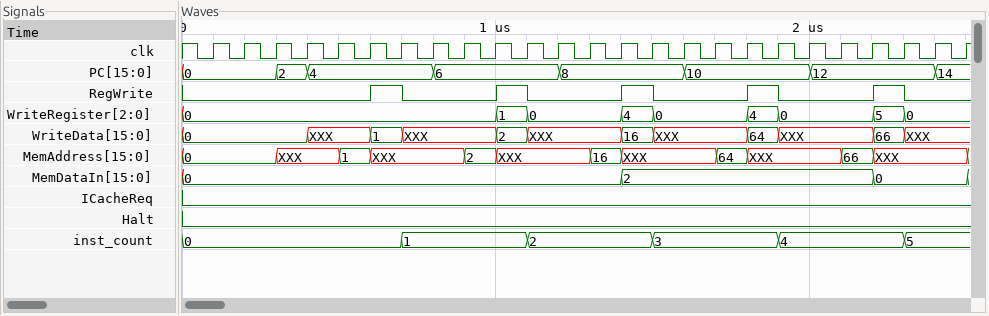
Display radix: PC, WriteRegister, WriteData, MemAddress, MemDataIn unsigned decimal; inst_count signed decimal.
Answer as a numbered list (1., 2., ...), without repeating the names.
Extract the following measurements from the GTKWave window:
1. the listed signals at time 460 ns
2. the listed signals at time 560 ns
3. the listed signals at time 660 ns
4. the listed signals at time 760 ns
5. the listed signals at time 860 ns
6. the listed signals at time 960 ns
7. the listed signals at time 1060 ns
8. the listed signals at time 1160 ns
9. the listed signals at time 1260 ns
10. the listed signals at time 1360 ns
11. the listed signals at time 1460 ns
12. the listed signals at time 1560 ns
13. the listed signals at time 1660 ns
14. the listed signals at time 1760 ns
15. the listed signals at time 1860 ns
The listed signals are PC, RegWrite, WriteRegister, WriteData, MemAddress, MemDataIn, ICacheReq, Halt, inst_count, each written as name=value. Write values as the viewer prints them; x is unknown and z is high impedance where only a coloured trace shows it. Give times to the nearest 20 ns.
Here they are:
1. PC=4, RegWrite=0, WriteRegister=0, WriteData=XXX, MemAddress=XXX, MemDataIn=0, ICacheReq=0, Halt=0, inst_count=0
2. PC=4, RegWrite=0, WriteRegister=0, WriteData=XXX, MemAddress=1, MemDataIn=0, ICacheReq=0, Halt=0, inst_count=0
3. PC=4, RegWrite=1, WriteRegister=0, WriteData=1, MemAddress=XXX, MemDataIn=0, ICacheReq=0, Halt=0, inst_count=0
4. PC=4, RegWrite=0, WriteRegister=0, WriteData=XXX, MemAddress=XXX, MemDataIn=0, ICacheReq=0, Halt=0, inst_count=1
5. PC=6, RegWrite=0, WriteRegister=0, WriteData=XXX, MemAddress=XXX, MemDataIn=0, ICacheReq=0, Halt=0, inst_count=1
6. PC=6, RegWrite=0, WriteRegister=0, WriteData=XXX, MemAddress=2, MemDataIn=0, ICacheReq=0, Halt=0, inst_count=1
7. PC=6, RegWrite=1, WriteRegister=1, WriteData=2, MemAddress=XXX, MemDataIn=0, ICacheReq=0, Halt=0, inst_count=1
8. PC=6, RegWrite=0, WriteRegister=0, WriteData=XXX, MemAddress=XXX, MemDataIn=0, ICacheReq=0, Halt=0, inst_count=2
9. PC=8, RegWrite=0, WriteRegister=0, WriteData=XXX, MemAddress=XXX, MemDataIn=0, ICacheReq=0, Halt=0, inst_count=2
10. PC=8, RegWrite=0, WriteRegister=0, WriteData=XXX, MemAddress=16, MemDataIn=0, ICacheReq=0, Halt=0, inst_count=2
11. PC=8, RegWrite=1, WriteRegister=4, WriteData=16, MemAddress=XXX, MemDataIn=2, ICacheReq=0, Halt=0, inst_count=2
12. PC=8, RegWrite=0, WriteRegister=0, WriteData=XXX, MemAddress=XXX, MemDataIn=2, ICacheReq=0, Halt=0, inst_count=3
13. PC=10, RegWrite=0, WriteRegister=0, WriteData=XXX, MemAddress=XXX, MemDataIn=2, ICacheReq=0, Halt=0, inst_count=3
14. PC=10, RegWrite=0, WriteRegister=0, WriteData=XXX, MemAddress=64, MemDataIn=2, ICacheReq=0, Halt=0, inst_count=3
15. PC=10, RegWrite=1, WriteRegister=4, WriteData=64, MemAddress=XXX, MemDataIn=2, ICacheReq=0, Halt=0, inst_count=3
